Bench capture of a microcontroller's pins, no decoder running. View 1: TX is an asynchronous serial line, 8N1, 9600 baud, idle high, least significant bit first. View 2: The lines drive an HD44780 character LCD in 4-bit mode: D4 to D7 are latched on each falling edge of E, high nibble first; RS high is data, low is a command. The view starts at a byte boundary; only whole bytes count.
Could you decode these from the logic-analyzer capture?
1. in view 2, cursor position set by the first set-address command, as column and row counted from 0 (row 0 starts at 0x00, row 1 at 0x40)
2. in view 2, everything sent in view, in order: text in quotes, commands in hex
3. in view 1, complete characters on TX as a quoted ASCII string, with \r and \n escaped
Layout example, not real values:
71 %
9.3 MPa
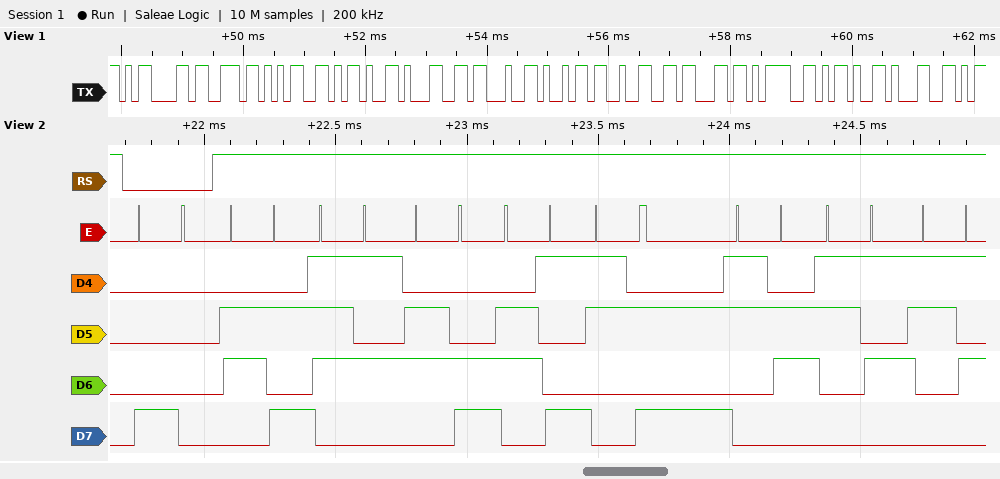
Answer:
column 0, row 0
0x80 "juli:655"
"\rs5-1#i2c=-1"
